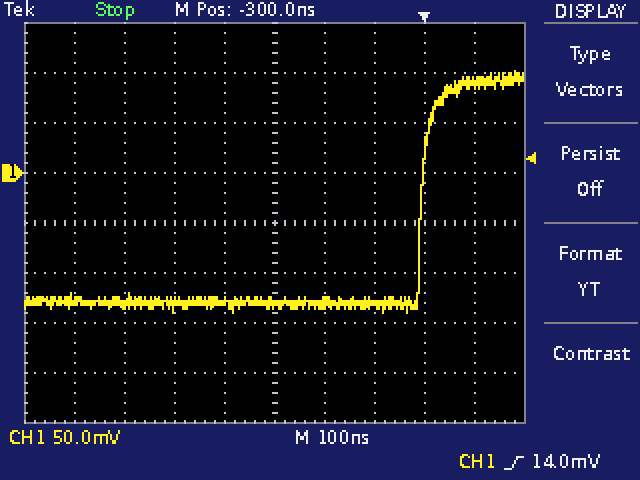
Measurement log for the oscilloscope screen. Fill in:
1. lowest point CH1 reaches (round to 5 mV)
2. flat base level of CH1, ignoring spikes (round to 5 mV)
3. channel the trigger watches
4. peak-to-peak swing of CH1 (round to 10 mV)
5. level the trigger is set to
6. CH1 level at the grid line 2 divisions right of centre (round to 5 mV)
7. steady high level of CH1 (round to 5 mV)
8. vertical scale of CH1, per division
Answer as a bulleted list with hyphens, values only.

- -140 mV
- -130 mV
- CH1
- 240 mV
- 14.0 mV
- -130 mV
- 90 mV
- 50 mV
